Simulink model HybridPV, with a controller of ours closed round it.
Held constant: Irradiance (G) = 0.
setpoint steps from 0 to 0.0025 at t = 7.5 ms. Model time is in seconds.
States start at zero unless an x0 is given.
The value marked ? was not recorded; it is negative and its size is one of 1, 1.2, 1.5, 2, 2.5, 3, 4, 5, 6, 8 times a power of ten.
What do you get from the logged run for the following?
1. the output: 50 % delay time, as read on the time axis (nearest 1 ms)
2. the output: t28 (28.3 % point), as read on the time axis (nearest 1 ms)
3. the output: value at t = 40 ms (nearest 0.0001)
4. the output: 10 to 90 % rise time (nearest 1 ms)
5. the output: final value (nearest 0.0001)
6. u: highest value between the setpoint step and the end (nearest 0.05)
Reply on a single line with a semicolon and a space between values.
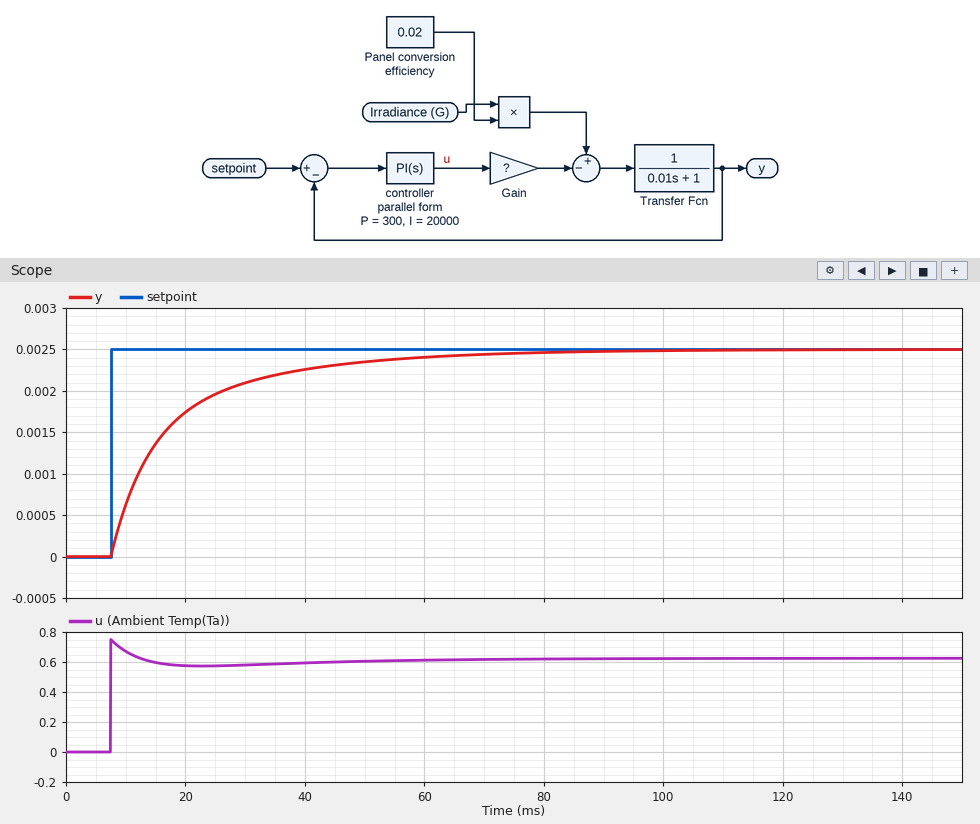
14 ms; 10 ms; 0.0023; 31 ms; 0.0025; 0.75
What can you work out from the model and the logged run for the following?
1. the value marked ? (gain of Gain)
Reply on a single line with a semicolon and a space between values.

-0.004
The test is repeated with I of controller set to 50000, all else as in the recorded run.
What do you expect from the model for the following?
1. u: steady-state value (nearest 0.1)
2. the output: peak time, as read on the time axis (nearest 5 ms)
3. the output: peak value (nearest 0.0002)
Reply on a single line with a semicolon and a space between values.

0.6; 30 ms; 0.0026
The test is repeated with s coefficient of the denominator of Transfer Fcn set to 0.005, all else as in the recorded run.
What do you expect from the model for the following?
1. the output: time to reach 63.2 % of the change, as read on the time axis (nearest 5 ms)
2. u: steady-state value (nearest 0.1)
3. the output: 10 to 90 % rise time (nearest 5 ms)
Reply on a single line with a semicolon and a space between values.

15 ms; 0.6; 35 ms
